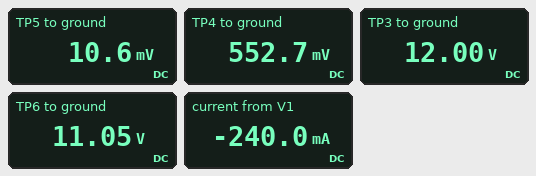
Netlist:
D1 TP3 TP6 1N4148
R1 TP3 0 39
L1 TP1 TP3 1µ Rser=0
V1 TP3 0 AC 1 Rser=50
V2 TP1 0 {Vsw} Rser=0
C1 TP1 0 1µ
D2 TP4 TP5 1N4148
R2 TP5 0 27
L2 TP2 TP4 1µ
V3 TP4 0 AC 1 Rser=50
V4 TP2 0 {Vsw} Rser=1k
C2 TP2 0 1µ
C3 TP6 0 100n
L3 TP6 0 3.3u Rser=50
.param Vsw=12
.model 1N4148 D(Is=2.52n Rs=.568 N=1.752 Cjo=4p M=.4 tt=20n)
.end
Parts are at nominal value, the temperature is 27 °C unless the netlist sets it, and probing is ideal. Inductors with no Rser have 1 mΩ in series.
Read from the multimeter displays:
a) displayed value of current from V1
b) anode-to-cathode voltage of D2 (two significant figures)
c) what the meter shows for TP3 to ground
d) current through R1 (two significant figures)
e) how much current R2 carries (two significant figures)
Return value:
-240.0 mA
540 mV
12.00 V
310 mA
390 µA
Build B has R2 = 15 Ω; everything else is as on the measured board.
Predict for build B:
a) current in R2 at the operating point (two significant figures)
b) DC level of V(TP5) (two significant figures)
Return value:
420 µA
6.3 mV
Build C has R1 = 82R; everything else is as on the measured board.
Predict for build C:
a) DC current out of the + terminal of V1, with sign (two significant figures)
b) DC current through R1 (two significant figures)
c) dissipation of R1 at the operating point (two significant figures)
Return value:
-240 mA
150 mA
1.8 W
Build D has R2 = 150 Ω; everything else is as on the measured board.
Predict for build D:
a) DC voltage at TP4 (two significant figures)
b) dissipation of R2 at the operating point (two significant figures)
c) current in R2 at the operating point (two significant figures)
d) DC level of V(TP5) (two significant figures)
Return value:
560 mV
9.5 µW
250 µA
38 mV
